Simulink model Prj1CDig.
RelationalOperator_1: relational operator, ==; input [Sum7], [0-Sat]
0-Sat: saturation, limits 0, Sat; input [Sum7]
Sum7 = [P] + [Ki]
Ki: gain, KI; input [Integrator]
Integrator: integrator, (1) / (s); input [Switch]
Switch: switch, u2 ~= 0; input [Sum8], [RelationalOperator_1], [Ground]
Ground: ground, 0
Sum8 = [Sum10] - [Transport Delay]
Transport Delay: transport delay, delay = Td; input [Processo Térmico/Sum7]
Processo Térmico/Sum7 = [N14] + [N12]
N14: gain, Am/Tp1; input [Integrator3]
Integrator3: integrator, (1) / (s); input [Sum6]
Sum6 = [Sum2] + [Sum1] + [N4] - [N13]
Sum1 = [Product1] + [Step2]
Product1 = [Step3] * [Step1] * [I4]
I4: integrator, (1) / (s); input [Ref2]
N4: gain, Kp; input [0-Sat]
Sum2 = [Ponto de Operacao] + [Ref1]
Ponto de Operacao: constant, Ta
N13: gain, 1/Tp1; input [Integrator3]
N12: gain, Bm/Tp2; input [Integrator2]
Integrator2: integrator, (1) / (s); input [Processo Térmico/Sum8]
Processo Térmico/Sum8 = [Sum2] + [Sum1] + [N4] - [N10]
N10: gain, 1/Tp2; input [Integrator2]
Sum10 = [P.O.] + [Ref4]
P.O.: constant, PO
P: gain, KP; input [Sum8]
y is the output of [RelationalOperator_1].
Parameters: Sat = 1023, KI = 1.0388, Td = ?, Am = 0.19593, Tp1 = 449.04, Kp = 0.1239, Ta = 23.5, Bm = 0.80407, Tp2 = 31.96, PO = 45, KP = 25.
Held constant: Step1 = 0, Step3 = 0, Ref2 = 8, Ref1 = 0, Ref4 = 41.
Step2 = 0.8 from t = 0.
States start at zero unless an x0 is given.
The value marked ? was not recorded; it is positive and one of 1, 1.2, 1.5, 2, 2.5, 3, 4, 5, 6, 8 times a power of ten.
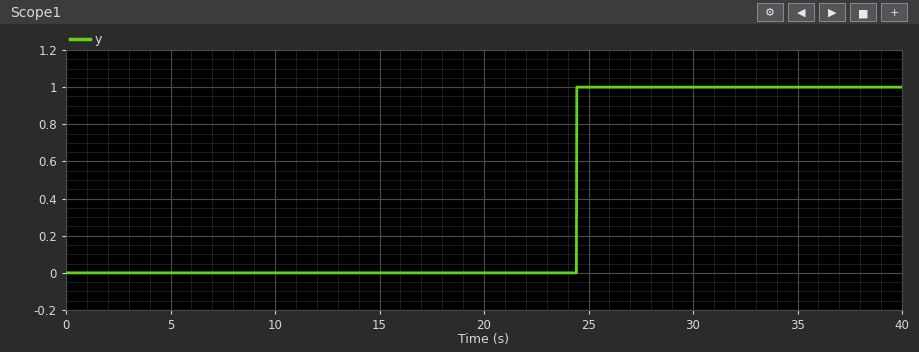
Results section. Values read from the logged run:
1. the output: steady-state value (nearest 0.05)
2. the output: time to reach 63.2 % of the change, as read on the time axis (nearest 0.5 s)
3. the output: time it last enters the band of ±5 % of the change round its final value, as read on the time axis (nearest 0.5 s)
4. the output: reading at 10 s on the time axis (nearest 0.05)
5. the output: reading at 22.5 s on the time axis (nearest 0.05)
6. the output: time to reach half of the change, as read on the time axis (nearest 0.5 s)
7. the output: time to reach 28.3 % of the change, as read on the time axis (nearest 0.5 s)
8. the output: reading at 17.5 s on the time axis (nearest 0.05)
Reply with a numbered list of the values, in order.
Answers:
1. 1.00
2. 24.5 s
3. 24.5 s
4. 0.00
5. 0.00
6. 24.5 s
7. 24.5 s
8. 0.00
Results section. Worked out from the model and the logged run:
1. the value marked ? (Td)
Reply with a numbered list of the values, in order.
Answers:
1. 10
